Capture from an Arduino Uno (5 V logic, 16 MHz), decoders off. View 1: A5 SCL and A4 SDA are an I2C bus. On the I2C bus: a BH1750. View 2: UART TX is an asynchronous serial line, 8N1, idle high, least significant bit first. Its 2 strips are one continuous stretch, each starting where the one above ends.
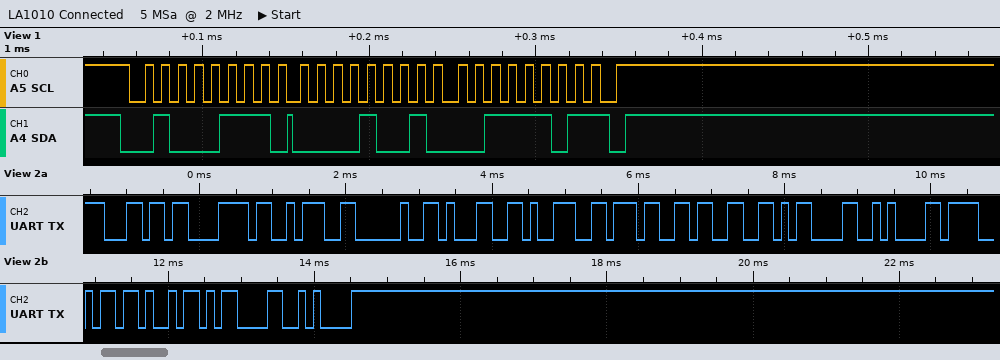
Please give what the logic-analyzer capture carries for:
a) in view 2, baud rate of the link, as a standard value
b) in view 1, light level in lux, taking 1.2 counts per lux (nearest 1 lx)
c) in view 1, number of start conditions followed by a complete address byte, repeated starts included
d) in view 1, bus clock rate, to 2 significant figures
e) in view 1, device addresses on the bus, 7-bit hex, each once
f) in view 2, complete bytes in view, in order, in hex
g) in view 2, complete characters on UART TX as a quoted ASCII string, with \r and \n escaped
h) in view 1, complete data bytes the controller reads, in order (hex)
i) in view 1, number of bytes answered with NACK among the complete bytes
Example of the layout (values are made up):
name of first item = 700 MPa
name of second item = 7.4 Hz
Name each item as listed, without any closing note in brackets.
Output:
in view 2, baud rate of the link, as a standard value = 9600 baud
in view 1, light level in lux, taking 1.2 counts per lux = 1971 lx
in view 1, number of start conditions followed by a complete address byte, repeated starts included = 1
in view 1, bus clock rate, to 2 significant figures = 100 kHz
in view 1, device addresses on the bus, 7-bit hex, each once = 0x23
in view 2, complete bytes in view, in order, in hex = 6C 78 3A 20 31 39 37 33 0D 0A 4F 4B 0D 0A
in view 2, complete characters on UART TX as a quoted ASCII string, with \r and \n escaped = "lx: 1973\r\nOK\r\n"
in view 1, complete data bytes the controller reads, in order = 09 3D
in view 1, number of bytes answered with NACK among the complete bytes = 1
